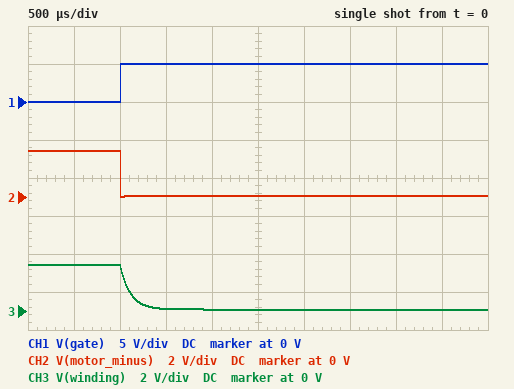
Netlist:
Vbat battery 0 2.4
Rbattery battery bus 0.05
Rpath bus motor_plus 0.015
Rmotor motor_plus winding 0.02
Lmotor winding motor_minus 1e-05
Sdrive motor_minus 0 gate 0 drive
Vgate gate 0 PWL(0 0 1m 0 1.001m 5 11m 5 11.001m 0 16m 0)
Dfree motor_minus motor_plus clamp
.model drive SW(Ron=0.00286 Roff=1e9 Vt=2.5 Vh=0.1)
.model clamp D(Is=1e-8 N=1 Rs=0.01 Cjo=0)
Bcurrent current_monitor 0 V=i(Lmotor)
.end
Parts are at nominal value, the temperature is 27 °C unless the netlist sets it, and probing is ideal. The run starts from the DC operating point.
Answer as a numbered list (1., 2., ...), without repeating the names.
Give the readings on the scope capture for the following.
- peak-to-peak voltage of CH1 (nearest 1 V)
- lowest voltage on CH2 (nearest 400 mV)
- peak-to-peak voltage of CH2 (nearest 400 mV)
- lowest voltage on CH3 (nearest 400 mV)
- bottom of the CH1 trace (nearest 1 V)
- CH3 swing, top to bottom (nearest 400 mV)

1. 5 V
2. 0 V
3. 2.4 V
4. 0 V
5. 0 V
6. 2.4 V
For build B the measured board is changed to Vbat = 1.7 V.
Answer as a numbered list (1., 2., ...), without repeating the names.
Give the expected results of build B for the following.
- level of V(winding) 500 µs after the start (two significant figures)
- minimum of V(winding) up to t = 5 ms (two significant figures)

1. 1.7 V
2. 55 mV
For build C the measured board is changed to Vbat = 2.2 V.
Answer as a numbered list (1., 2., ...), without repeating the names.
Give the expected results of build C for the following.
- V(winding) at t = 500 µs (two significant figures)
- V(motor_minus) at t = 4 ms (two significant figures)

1. 2.2 V
2. 72 mV
